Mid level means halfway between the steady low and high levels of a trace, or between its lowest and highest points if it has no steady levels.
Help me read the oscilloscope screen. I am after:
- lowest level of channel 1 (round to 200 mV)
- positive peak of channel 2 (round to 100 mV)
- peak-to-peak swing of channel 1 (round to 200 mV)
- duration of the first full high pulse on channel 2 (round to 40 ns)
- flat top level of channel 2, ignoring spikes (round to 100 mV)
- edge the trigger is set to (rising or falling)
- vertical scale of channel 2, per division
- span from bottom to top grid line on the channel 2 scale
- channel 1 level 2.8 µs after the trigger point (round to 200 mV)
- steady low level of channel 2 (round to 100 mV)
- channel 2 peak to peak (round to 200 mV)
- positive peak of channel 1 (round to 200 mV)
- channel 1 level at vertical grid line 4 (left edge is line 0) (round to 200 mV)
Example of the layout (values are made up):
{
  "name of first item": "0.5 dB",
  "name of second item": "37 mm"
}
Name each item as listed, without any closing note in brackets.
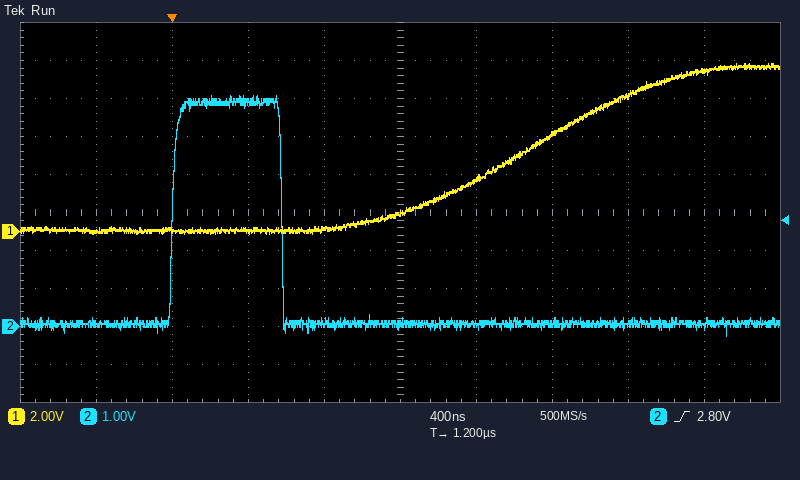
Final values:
{
  "lowest level of channel 1": "-200 mV",
  "positive peak of channel 2": "6.1 V",
  "peak-to-peak swing of channel 1": "9.0 V",
  "duration of the first full high pulse on channel 2": "560 ns",
  "flat top level of channel 2, ignoring spikes": "5.9 V",
  "edge the trigger is set to": "rising",
  "vertical scale of channel 2, per division": "1 V",
  "span from bottom to top grid line on the channel 2 scale": "10 V",
  "channel 1 level 2.8 µs after the trigger point": "8.4 V",
  "steady low level of channel 2": "100 mV",
  "channel 2 peak to peak": "6.4 V",
  "positive peak of channel 1": "8.8 V",
  "channel 1 level at vertical grid line 4 (left edge is line 0)": "200 mV"
}
